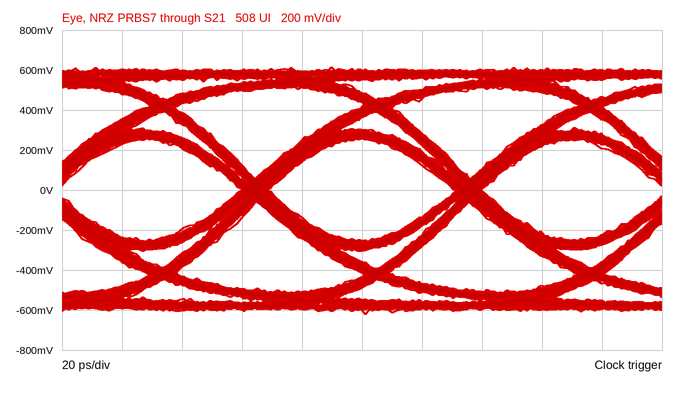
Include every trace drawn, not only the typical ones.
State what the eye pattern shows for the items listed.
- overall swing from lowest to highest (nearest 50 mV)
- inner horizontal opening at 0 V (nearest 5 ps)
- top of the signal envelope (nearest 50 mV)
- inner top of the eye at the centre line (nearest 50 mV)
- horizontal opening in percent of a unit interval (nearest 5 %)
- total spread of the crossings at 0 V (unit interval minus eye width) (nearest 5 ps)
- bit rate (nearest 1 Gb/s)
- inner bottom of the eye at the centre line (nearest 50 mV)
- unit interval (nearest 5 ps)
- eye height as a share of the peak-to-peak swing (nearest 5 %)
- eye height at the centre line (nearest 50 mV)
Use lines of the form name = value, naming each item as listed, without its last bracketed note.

overall swing from lowest to highest = 1.25 V
inner horizontal opening at 0 V = 60 ps
top of the signal envelope = 600 mV
inner top of the eye at the centre line = 250 mV
horizontal opening in percent of a unit interval = 85 %
total spread of the crossings at 0 V (unit interval minus eye width) = 10 ps
bit rate = 14 Gb/s
inner bottom of the eye at the centre line = -250 mV
unit interval = 70 ps
eye height as a share of the peak-to-peak swing = 40 %
eye height at the centre line = 500 mV
